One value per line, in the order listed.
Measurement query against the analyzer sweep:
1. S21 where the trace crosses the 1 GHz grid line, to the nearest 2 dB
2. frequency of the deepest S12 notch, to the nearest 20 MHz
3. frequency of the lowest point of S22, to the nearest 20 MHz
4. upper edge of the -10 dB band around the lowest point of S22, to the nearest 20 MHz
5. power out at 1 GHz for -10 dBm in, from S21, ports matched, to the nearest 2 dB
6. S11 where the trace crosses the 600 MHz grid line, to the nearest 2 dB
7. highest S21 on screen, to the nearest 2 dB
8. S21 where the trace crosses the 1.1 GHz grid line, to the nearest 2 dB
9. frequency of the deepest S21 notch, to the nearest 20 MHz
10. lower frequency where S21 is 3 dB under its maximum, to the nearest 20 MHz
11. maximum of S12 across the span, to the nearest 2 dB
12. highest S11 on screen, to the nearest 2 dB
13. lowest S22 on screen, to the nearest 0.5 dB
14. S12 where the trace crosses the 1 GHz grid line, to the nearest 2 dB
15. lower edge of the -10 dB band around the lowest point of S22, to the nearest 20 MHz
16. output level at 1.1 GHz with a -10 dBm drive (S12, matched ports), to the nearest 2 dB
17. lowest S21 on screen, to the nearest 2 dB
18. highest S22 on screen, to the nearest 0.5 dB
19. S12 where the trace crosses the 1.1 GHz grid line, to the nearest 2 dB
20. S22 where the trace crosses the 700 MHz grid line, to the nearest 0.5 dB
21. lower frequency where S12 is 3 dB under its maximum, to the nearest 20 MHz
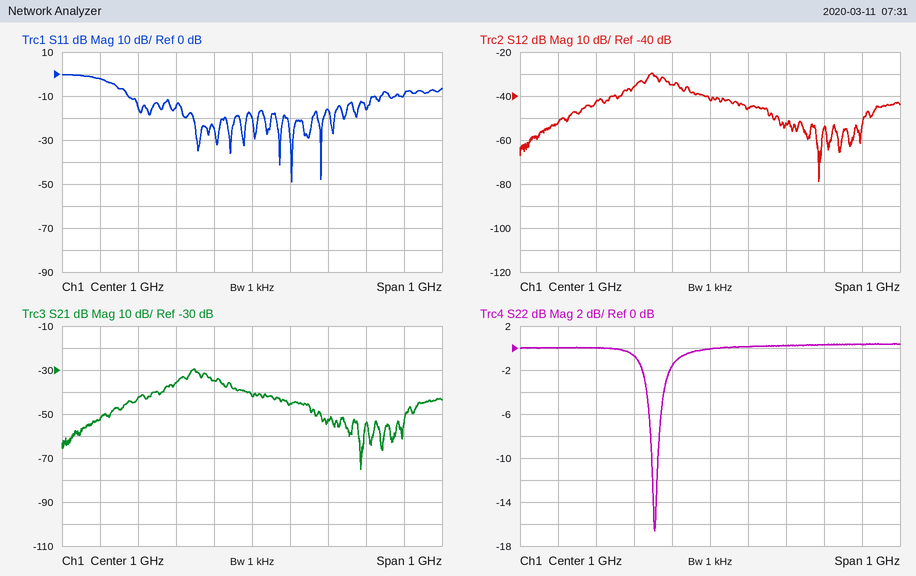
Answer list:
-42 dB
1.28 GHz
860 MHz
860 MHz
-52 dBm
-2 dB
-30 dB
-46 dB
1.28 GHz
840 MHz
-30 dB
0 dB
-16.5 dB
-42 dB
840 MHz
-56 dBm
-76 dB
0.5 dB
-46 dB
0.0 dB
840 MHz
